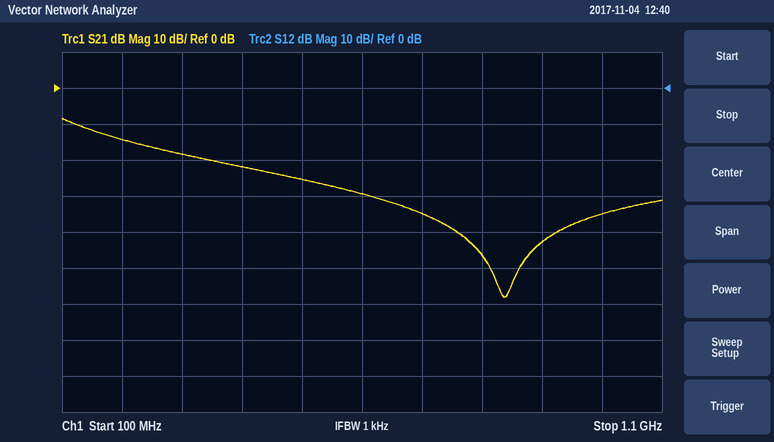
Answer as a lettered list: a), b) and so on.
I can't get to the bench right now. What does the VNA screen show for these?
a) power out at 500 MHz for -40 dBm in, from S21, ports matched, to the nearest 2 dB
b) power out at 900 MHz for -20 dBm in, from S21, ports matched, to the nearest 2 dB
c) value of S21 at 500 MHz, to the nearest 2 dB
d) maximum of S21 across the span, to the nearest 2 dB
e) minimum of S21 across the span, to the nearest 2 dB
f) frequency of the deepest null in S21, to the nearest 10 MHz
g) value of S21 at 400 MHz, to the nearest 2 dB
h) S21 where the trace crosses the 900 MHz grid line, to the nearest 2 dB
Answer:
a) -66 dBm
b) -62 dBm
c) -26 dB
d) -8 dB
e) -58 dB
f) 840 MHz
g) -22 dB
h) -42 dB
